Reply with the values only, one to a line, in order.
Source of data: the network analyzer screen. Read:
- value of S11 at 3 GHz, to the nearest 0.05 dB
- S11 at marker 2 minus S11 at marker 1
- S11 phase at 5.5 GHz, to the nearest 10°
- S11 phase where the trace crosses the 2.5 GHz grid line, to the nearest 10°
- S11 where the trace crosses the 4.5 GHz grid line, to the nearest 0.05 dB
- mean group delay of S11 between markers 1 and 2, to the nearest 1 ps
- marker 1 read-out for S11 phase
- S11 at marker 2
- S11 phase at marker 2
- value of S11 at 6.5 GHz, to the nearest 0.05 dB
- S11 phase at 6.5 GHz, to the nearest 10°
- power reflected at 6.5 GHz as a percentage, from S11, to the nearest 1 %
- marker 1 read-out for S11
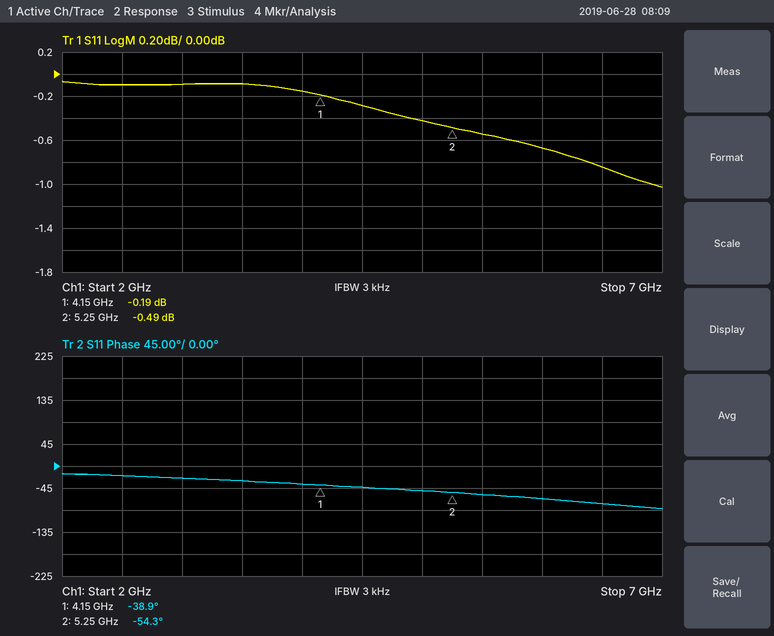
-0.10 dB
-0.30 dB
-60°
-20°
-0.30 dB
39 ps
-38.9°
-0.49 dB
-54.3°
-0.85 dB
-80°
82 %
-0.19 dB
